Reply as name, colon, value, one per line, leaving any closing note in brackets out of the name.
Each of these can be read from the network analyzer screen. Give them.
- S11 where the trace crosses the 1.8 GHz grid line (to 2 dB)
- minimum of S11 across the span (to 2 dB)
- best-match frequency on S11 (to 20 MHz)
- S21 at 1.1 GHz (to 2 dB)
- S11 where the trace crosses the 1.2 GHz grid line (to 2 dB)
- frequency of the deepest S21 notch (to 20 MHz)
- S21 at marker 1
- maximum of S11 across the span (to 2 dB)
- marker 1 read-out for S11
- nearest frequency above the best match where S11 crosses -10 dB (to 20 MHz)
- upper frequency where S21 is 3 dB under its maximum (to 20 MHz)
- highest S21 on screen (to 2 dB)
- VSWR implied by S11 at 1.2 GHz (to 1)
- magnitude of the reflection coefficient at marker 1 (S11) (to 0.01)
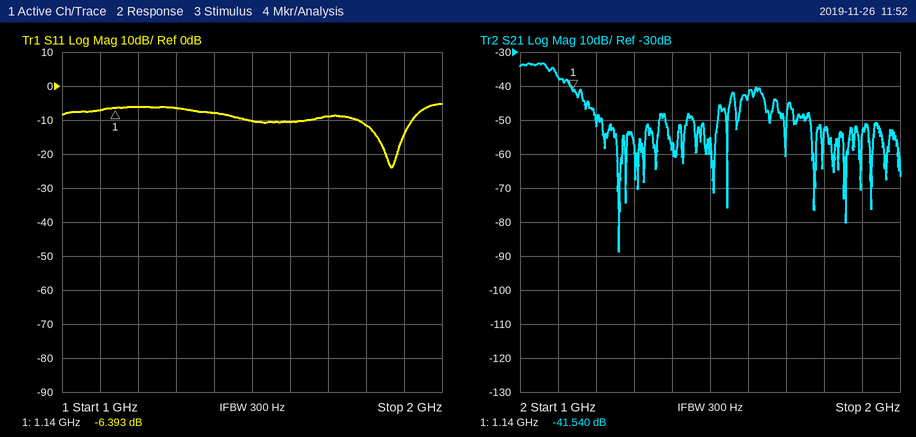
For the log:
S11 where the trace crosses the 1.8 GHz grid line: -12 dB
minimum of S11 across the span: -24 dB
best-match frequency on S11: 1.86 GHz
S21 at 1.1 GHz: -38 dB
S11 where the trace crosses the 1.2 GHz grid line: -6 dB
frequency of the deepest S21 notch: 1.26 GHz
S21 at marker 1: -41.540 dB
maximum of S11 across the span: -6 dB
marker 1 read-out for S11: -6.393 dB
nearest frequency above the best match where S11 crosses -10 dB: 1.92 GHz
upper frequency where S21 is 3 dB under its maximum: 1.10 GHz
highest S21 on screen: -34 dB
VSWR implied by S11 at 1.2 GHz: 3
magnitude of the reflection coefficient at marker 1 (S11): 0.48
